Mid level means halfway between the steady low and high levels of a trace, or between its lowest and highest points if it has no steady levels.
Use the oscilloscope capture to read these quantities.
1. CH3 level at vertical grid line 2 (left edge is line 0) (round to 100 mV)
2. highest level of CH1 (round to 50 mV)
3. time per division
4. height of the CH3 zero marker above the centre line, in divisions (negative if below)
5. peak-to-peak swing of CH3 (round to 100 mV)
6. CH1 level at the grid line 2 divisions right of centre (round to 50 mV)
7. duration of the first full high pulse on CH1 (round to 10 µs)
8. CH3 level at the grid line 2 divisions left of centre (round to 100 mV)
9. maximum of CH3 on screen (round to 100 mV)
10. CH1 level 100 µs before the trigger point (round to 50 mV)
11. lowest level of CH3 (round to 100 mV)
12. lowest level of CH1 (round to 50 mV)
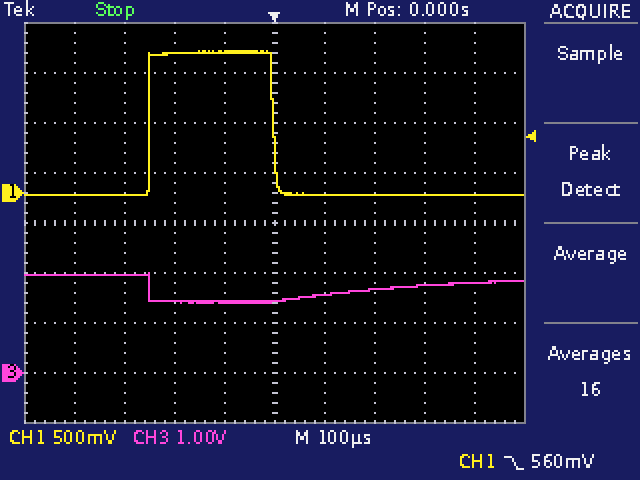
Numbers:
2.0 V
1.40 V
100 µs
-3.0 div
600 mV
0 mV
250 µs
1.4 V
2.0 V
1.40 V
1.4 V
0 mV
